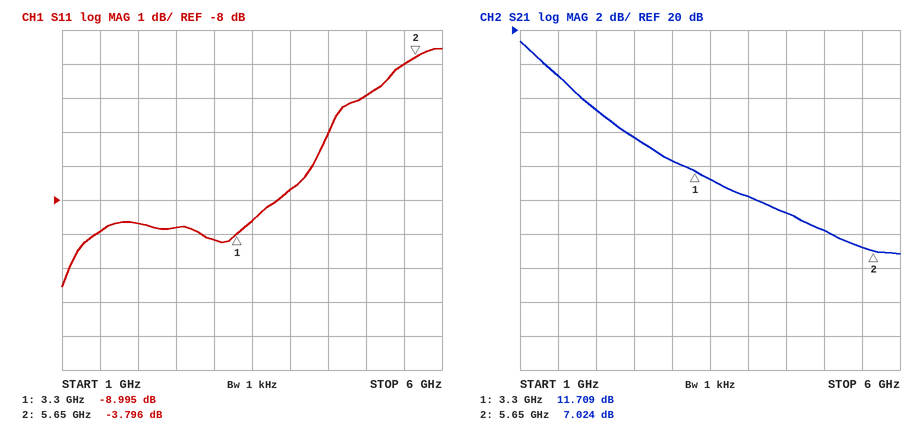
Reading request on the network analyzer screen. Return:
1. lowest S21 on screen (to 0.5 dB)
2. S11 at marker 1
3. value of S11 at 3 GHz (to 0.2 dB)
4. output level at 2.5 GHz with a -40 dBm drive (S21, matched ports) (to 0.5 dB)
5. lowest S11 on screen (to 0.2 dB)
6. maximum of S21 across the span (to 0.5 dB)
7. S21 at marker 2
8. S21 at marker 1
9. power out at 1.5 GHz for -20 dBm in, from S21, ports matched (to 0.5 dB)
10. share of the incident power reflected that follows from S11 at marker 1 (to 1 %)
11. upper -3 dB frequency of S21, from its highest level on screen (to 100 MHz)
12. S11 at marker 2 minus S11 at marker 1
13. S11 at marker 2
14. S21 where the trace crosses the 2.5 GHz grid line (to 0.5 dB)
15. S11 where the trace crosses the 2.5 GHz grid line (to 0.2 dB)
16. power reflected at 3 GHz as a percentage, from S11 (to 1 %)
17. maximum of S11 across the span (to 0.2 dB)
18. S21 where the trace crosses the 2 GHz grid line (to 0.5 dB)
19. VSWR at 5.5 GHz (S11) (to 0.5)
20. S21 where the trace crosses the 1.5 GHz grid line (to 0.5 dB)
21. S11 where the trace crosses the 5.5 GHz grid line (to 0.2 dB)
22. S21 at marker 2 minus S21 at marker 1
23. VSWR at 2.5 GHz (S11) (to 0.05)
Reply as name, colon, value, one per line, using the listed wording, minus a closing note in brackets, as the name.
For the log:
lowest S21 on screen: 7.0 dB
S11 at marker 1: -8.995 dB
value of S11 at 3 GHz: -9.2 dB
output level at 2.5 GHz with a -40 dBm drive (S21, matched ports): -26.5 dBm
lowest S11 on screen: -10.6 dB
maximum of S21 across the span: 19.5 dB
S21 at marker 2: 7.024 dB
S21 at marker 1: 11.709 dB
power out at 1.5 GHz for -20 dBm in, from S21, ports matched: -2.5 dBm
share of the incident power reflected that follows from S11 at marker 1: 13 %
upper -3 dB frequency of S21, from its highest level on screen: 1.7 GHz
S11 at marker 2 minus S11 at marker 1: 5.199 dB
S11 at marker 2: -3.796 dB
S21 where the trace crosses the 2.5 GHz grid line: 13.5 dB
S11 where the trace crosses the 2.5 GHz grid line: -8.8 dB
power reflected at 3 GHz as a percentage, from S11: 12 %
maximum of S11 across the span: -3.6 dB
S21 where the trace crosses the 2 GHz grid line: 15.5 dB
VSWR at 5.5 GHz (S11): 4.5
S21 where the trace crosses the 1.5 GHz grid line: 17.5 dB
S11 where the trace crosses the 5.5 GHz grid line: -4.0 dB
S21 at marker 2 minus S21 at marker 1: -4.685 dB
VSWR at 2.5 GHz (S11): 2.15
